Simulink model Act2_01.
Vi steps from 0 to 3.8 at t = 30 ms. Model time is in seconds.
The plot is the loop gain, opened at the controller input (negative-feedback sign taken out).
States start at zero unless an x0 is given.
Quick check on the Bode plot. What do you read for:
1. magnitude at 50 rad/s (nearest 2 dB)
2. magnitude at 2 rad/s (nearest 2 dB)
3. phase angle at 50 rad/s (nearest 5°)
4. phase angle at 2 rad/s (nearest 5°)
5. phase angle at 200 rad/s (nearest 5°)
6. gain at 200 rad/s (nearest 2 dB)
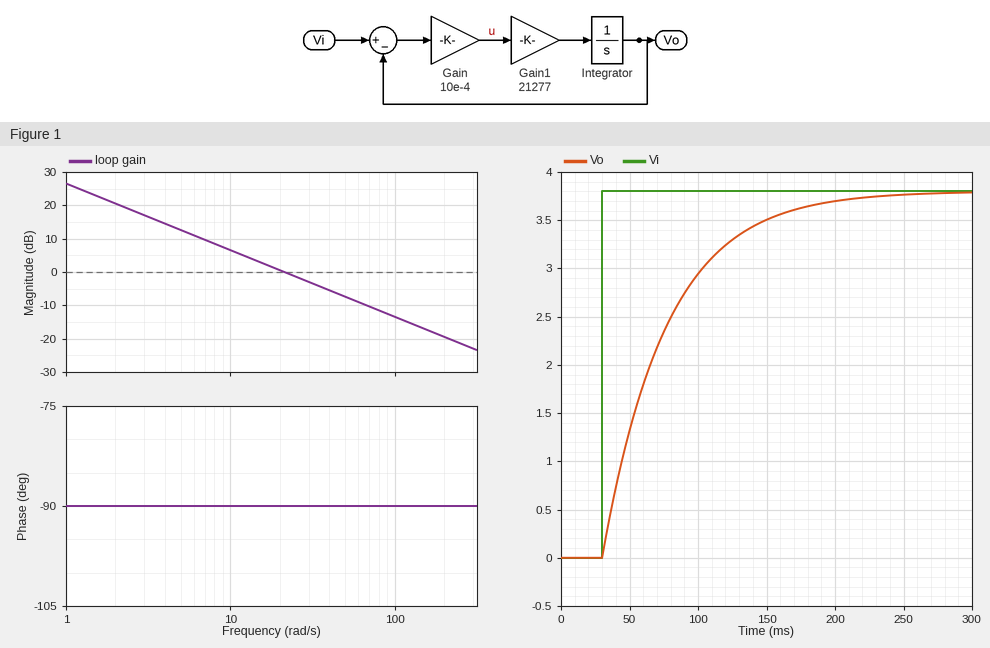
-8 dB
20 dB
-90°
-90°
-90°
-20 dB
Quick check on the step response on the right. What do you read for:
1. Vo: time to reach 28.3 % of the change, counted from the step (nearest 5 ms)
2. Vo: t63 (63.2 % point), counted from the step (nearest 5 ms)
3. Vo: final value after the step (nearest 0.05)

15 ms
45 ms
3.80
